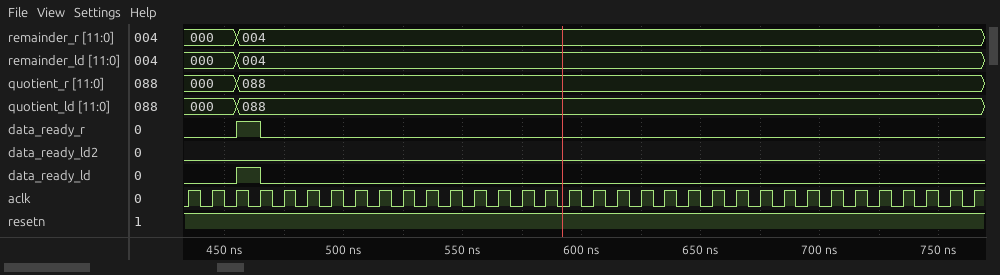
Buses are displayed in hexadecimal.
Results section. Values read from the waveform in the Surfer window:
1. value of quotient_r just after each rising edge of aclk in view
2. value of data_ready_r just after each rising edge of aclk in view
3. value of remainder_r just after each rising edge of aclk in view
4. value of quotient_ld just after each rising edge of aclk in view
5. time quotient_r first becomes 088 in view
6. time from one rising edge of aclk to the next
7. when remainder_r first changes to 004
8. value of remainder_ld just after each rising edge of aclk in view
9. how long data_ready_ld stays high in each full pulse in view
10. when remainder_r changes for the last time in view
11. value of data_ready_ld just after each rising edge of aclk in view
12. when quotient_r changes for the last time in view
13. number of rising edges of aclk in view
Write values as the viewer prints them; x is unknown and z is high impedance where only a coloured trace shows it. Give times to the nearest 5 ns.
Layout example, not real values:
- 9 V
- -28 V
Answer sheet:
- 000, 000, 088, 088, 088, 088, 088, 088, 088, 088, 088, 088, 088, 088, 088, 088, 088, 088, 088, 088, 088, 088, 088, 088, 088, 088, 088, 088, 088, 088, 088, 088, 088, 088
- 0 0 1 0 0 0 0 0 0 0 0 0 0 0 0 0 0 0 0 0 0 0 0 0 0 0 0 0 0 0 0 0 0 0
- 000, 000, 004, 004, 004, 004, 004, 004, 004, 004, 004, 004, 004, 004, 004, 004, 004, 004, 004, 004, 004, 004, 004, 004, 004, 004, 004, 004, 004, 004, 004, 004, 004, 004
- 000, 000, 088, 088, 088, 088, 088, 088, 088, 088, 088, 088, 088, 088, 088, 088, 088, 088, 088, 088, 088, 088, 088, 088, 088, 088, 088, 088, 088, 088, 088, 088, 088, 088
- 455 ns
- 10 ns
- 455 ns
- 000, 000, 004, 004, 004, 004, 004, 004, 004, 004, 004, 004, 004, 004, 004, 004, 004, 004, 004, 004, 004, 004, 004, 004, 004, 004, 004, 004, 004, 004, 004, 004, 004, 004
- 10 ns
- 455 ns
- 0 0 1 0 0 0 0 0 0 0 0 0 0 0 0 0 0 0 0 0 0 0 0 0 0 0 0 0 0 0 0 0 0 0
- 455 ns
- 34
